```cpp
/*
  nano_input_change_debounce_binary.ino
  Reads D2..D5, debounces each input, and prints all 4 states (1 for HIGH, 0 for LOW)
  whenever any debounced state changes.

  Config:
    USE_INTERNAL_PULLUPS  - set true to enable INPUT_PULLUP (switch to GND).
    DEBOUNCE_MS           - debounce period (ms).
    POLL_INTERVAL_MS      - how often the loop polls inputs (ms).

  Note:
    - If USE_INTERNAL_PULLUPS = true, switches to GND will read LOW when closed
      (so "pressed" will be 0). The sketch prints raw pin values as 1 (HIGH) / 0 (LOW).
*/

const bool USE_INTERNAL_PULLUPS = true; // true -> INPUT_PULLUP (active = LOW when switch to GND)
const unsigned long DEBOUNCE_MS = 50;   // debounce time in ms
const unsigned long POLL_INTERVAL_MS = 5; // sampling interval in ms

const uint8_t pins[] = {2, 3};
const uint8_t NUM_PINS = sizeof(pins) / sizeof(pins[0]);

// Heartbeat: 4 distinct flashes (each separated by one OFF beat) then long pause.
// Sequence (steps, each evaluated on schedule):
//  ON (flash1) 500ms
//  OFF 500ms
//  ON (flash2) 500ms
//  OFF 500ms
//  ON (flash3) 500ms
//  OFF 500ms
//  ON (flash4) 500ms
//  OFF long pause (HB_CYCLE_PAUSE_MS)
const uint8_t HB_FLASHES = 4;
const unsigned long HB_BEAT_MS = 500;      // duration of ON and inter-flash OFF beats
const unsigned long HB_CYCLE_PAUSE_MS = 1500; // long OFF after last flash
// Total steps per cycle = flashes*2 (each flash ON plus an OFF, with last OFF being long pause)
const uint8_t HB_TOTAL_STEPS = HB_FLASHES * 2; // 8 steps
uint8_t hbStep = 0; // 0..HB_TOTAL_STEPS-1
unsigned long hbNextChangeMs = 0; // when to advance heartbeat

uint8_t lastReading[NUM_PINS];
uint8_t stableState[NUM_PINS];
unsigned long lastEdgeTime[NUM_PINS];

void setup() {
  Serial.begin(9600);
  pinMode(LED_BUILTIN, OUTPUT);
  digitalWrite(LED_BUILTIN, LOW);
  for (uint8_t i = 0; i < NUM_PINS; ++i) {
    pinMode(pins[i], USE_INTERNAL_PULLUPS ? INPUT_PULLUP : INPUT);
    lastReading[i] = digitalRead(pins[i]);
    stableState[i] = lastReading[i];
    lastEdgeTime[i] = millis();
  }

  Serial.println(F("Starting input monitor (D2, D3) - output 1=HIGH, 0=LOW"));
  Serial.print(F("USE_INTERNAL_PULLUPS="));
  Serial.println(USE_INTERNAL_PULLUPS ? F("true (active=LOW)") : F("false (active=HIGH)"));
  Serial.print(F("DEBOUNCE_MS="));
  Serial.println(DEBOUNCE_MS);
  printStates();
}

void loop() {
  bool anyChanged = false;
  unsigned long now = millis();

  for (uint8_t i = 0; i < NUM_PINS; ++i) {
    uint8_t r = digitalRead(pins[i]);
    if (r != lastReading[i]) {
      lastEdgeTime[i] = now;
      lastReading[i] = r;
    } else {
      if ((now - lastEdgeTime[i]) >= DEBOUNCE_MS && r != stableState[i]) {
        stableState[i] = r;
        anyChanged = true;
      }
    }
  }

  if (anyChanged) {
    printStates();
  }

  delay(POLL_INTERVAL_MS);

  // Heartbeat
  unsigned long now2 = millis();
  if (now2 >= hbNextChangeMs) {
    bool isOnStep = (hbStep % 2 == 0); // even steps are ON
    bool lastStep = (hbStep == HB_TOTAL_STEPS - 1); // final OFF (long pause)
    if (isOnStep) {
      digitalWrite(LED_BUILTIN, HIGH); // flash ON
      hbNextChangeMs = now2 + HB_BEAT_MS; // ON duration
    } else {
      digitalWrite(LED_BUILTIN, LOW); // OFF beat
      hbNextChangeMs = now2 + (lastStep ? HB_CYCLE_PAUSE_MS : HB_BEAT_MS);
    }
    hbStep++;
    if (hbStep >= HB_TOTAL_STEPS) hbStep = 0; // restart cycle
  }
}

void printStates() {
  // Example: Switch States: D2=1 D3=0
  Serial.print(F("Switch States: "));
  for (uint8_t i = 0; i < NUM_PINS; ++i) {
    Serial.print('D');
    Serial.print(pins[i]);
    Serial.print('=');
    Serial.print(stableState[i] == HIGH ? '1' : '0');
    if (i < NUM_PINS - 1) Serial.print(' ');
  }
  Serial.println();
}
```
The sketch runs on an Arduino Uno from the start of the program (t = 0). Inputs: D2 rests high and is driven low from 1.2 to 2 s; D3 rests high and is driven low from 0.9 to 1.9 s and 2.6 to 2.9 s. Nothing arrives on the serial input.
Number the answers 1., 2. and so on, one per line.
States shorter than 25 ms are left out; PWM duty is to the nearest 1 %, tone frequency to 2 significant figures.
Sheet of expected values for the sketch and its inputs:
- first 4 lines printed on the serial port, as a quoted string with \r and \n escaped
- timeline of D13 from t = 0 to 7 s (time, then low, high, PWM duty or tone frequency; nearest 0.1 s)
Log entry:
1. "Starting input monitor (D2, D3) - output 1=HIGH, 0=LOW\r\nUSE_INTERNAL_PULLUPS=true (active=LOW)\r\nDEBOUNCE_MS=50\r\nSwitch States: D2=1 D3=1\r\n"
2. 0 s low; 0.1 s high; 0.6 s low; 1.1 s high; 1.6 s low; 2.1 s high; 2.6 s low; 3.1 s high; 3.6 s low; 5.1 s high; 5.6 s low; 6.1 s high; 6.6 s low
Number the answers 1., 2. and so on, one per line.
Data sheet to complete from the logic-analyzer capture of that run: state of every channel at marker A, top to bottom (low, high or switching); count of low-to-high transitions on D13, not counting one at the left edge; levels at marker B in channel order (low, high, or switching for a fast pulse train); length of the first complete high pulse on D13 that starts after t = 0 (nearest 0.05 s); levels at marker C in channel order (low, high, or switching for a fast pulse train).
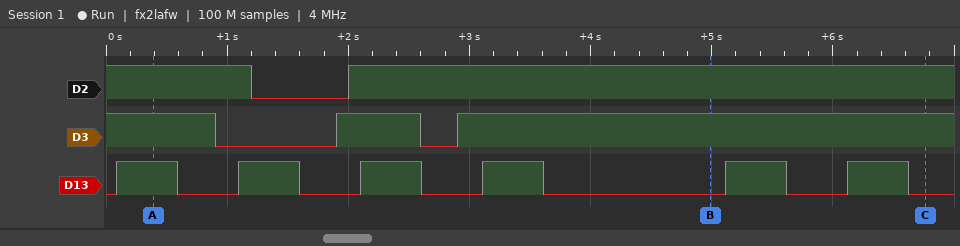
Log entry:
1. D2 high, D3 high, D13 high
2. 6
3. D2 high, D3 high, D13 low
4. 0.50 s
5. D2 high, D3 high, D13 low
